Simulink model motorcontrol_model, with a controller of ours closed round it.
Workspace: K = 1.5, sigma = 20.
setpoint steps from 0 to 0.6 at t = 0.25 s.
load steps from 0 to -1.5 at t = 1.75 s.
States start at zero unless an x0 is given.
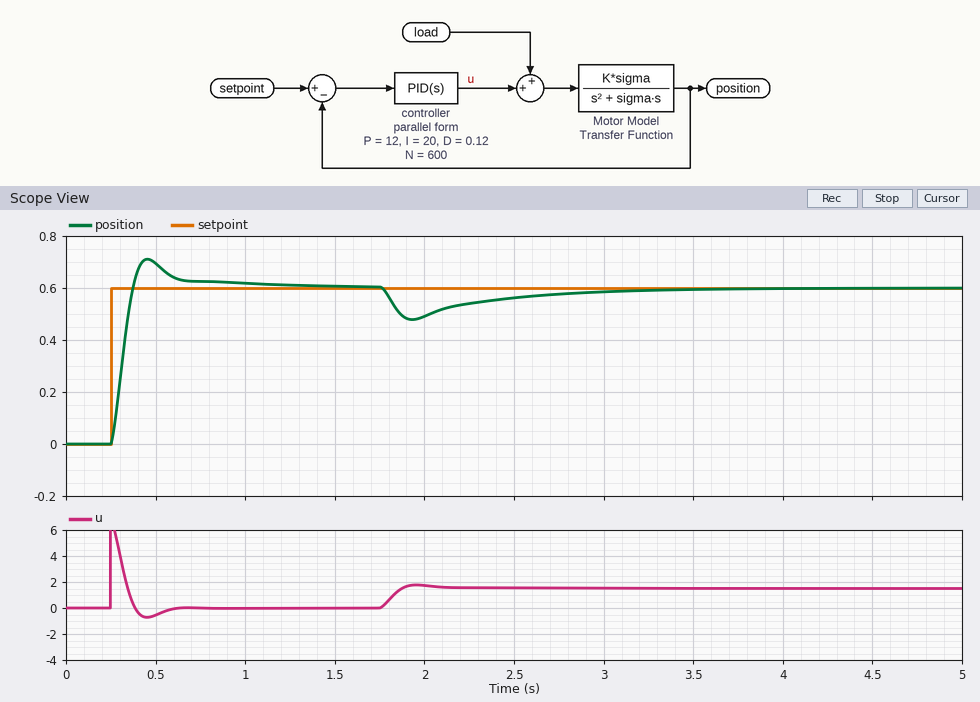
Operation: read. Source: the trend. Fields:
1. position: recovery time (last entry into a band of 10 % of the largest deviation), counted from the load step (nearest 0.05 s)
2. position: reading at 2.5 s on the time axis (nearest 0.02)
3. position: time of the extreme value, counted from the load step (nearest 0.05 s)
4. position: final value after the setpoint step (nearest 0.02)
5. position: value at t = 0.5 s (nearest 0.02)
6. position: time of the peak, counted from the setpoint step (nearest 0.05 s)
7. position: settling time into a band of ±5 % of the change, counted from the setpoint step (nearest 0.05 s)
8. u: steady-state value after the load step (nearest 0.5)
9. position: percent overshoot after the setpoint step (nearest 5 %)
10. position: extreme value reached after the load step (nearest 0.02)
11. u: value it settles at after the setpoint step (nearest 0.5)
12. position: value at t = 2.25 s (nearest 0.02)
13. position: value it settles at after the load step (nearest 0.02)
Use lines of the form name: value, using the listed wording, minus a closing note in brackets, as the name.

position: recovery time (last entry into a band of 10 % of the largest deviation), counted from the load step: 1.35 s
position: reading at 2.5 s on the time axis: 0.56
position: time of the extreme value, counted from the load step: 0.20 s
position: final value after the setpoint step: 0.60
position: value at t = 0.5 s: 0.70
position: time of the peak, counted from the setpoint step: 0.20 s
position: settling time into a band of ±5 % of the change, counted from the setpoint step: 0.40 s
u: steady-state value after the load step: 1.5
position: percent overshoot after the setpoint step: 20 %
position: extreme value reached after the load step: 0.48
u: value it settles at after the setpoint step: 0.0
position: value at t = 2.25 s: 0.54
position: value it settles at after the load step: 0.60
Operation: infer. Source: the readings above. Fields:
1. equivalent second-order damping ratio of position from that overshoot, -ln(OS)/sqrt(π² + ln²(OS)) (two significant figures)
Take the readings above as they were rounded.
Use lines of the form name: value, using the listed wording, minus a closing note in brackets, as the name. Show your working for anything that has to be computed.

equivalent second-order damping ratio of position from that overshoot, -ln(OS)/sqrt(π² + ln²(OS)): ln(0.2) = -1.609; 1.609 / sqrt(9.870 + 2.590) = 0.46
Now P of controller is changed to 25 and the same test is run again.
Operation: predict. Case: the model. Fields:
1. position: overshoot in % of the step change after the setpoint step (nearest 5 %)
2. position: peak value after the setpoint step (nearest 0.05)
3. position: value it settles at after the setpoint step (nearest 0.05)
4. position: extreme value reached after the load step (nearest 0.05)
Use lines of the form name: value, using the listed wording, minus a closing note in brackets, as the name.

position: overshoot in % of the step change after the setpoint step: 25 %
position: peak value after the setpoint step: 0.75
position: value it settles at after the setpoint step: 0.60
position: extreme value reached after the load step: 0.55
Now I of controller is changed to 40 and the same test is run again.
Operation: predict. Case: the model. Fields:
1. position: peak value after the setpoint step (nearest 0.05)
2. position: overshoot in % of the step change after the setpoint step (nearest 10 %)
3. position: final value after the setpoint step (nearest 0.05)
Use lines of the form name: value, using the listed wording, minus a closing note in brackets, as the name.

position: peak value after the setpoint step: 0.75
position: overshoot in % of the step change after the setpoint step: 30 %
position: final value after the setpoint step: 0.60
